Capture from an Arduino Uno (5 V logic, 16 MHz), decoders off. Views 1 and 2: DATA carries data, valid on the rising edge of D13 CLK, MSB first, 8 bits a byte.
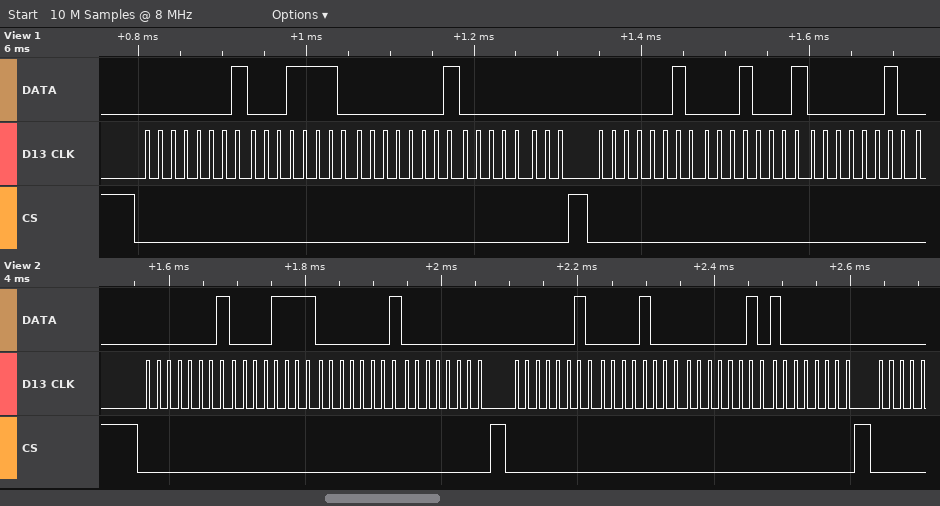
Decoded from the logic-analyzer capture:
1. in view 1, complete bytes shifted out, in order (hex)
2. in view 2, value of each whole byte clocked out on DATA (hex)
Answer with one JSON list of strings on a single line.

["01 1E 01 00 02 11 02", "0x01 0x0F 0x01 0x00 0x02 0x08 0x02 0x80"]
